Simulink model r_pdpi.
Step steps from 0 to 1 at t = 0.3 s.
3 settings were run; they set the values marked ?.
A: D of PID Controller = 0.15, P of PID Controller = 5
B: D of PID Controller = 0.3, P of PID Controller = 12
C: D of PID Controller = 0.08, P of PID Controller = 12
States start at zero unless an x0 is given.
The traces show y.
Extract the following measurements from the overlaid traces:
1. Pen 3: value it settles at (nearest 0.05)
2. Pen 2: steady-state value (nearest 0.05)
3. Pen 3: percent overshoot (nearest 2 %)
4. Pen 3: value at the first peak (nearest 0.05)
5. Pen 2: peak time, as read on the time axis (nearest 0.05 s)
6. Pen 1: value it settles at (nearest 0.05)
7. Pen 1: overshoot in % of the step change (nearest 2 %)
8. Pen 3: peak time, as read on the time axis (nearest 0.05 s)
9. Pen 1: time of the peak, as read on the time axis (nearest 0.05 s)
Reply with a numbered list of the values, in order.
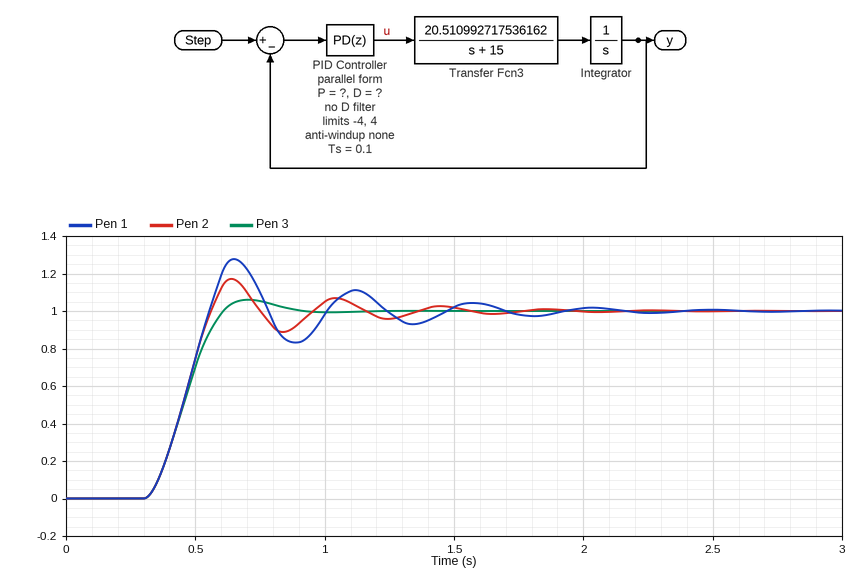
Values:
1. 1.00
2. 1.00
3. 6 %
4. 1.05
5. 0.65 s
6. 1.00
7. 28 %
8. 0.70 s
9. 0.65 s
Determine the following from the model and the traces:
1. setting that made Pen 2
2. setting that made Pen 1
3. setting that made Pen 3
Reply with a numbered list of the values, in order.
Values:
1. B
2. C
3. A
